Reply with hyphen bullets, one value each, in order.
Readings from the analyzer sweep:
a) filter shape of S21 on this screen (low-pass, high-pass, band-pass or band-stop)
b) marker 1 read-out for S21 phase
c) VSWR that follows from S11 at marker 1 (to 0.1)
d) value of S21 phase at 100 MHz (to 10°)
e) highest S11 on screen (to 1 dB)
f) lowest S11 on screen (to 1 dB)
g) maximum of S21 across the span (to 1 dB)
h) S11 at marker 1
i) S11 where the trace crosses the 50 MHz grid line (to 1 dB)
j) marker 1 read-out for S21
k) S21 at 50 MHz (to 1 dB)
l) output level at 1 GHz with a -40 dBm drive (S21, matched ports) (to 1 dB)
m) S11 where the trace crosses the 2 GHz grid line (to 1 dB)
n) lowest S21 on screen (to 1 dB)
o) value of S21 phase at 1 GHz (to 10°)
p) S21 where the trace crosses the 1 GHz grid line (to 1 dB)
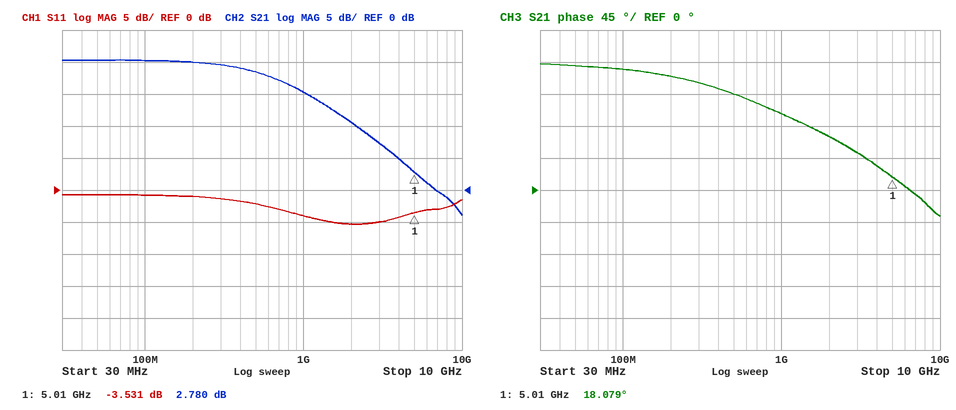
- low-pass
- 18.079°
- 5.0
- 170°
- -1 dB
- -5 dB
- 20 dB
- -3.531 dB
- -1 dB
- 2.780 dB
- 20 dB
- -25 dBm
- -5 dB
- -4 dB
- 110°
- 15 dB
